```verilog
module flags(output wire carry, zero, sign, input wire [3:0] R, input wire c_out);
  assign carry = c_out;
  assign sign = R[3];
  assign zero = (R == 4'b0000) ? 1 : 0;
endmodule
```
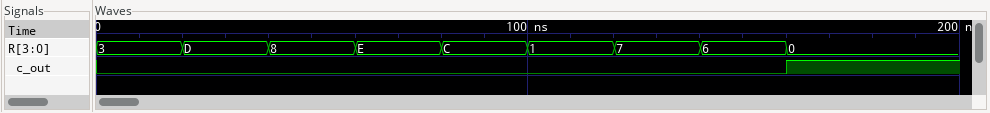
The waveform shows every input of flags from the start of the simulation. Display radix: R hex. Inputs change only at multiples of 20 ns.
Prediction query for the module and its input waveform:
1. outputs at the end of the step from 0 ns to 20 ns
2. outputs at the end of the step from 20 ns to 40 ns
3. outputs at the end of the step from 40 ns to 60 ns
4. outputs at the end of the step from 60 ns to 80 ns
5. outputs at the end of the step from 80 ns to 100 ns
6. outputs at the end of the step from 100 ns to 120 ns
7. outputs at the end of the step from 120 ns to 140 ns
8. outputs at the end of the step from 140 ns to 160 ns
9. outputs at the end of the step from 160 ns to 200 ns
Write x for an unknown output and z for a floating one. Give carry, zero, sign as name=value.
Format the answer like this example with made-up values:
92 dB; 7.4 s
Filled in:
carry=0, zero=0, sign=0; carry=0, zero=0, sign=1; carry=0, zero=0, sign=1; carry=0, zero=0, sign=1; carry=0, zero=0, sign=1; carry=0, zero=0, sign=0; carry=0, zero=0, sign=0; carry=0, zero=0, sign=0; carry=1, zero=1, sign=0
